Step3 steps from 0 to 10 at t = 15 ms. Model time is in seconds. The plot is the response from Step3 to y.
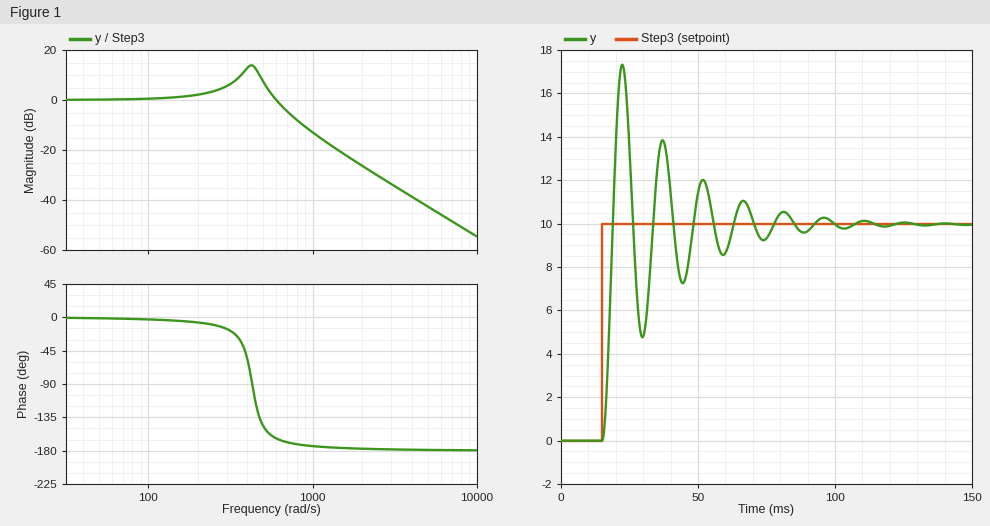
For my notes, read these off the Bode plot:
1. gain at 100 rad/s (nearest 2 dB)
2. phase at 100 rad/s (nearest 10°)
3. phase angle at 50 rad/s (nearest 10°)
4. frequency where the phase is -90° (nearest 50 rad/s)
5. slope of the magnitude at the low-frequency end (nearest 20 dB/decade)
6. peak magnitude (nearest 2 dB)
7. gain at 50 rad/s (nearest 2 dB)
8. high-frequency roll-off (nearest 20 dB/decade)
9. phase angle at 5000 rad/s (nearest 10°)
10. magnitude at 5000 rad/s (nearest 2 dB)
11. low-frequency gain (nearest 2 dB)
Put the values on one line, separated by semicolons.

0 dB; 0°; 0°; 450 rad/s; 0 dB/decade; 14 dB; 0 dB; -40 dB/decade; -180°; -42 dB; 0 dB
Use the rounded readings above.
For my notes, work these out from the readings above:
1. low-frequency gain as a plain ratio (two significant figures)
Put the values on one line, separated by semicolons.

1.0
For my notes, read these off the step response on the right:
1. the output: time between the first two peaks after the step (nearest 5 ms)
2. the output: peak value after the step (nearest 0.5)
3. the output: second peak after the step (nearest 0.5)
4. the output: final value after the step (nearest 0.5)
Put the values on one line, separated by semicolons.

15 ms; 17.5; 14.0; 10.0
